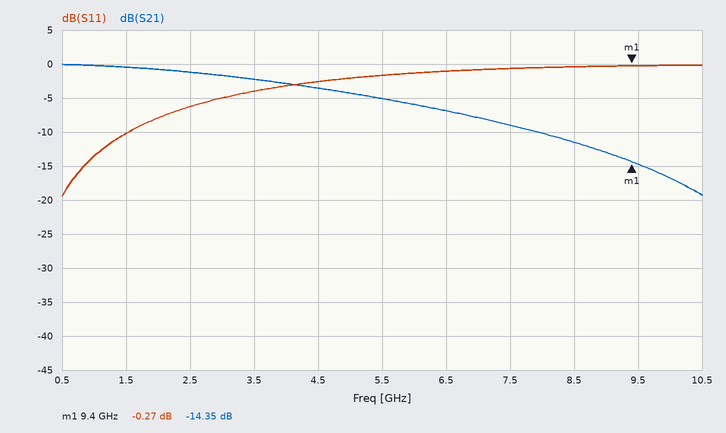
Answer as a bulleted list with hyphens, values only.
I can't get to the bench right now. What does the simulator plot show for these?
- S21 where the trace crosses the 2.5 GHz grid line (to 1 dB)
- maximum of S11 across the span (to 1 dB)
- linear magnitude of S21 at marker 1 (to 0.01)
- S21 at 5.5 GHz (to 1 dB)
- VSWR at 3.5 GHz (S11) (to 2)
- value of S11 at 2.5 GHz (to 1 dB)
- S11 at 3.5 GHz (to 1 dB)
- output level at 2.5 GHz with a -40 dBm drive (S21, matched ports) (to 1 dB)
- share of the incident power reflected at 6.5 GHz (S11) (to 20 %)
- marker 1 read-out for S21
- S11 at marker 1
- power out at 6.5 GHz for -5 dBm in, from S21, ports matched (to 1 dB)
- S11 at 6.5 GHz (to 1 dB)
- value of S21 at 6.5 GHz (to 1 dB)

- -1 dB
- 0 dB
- 0.19
- -5 dB
- 4
- -6 dB
- -4 dB
- -41 dBm
- 80 %
- -14.35 dB
- -0.27 dB
- -12 dBm
- -1 dB
- -7 dB
